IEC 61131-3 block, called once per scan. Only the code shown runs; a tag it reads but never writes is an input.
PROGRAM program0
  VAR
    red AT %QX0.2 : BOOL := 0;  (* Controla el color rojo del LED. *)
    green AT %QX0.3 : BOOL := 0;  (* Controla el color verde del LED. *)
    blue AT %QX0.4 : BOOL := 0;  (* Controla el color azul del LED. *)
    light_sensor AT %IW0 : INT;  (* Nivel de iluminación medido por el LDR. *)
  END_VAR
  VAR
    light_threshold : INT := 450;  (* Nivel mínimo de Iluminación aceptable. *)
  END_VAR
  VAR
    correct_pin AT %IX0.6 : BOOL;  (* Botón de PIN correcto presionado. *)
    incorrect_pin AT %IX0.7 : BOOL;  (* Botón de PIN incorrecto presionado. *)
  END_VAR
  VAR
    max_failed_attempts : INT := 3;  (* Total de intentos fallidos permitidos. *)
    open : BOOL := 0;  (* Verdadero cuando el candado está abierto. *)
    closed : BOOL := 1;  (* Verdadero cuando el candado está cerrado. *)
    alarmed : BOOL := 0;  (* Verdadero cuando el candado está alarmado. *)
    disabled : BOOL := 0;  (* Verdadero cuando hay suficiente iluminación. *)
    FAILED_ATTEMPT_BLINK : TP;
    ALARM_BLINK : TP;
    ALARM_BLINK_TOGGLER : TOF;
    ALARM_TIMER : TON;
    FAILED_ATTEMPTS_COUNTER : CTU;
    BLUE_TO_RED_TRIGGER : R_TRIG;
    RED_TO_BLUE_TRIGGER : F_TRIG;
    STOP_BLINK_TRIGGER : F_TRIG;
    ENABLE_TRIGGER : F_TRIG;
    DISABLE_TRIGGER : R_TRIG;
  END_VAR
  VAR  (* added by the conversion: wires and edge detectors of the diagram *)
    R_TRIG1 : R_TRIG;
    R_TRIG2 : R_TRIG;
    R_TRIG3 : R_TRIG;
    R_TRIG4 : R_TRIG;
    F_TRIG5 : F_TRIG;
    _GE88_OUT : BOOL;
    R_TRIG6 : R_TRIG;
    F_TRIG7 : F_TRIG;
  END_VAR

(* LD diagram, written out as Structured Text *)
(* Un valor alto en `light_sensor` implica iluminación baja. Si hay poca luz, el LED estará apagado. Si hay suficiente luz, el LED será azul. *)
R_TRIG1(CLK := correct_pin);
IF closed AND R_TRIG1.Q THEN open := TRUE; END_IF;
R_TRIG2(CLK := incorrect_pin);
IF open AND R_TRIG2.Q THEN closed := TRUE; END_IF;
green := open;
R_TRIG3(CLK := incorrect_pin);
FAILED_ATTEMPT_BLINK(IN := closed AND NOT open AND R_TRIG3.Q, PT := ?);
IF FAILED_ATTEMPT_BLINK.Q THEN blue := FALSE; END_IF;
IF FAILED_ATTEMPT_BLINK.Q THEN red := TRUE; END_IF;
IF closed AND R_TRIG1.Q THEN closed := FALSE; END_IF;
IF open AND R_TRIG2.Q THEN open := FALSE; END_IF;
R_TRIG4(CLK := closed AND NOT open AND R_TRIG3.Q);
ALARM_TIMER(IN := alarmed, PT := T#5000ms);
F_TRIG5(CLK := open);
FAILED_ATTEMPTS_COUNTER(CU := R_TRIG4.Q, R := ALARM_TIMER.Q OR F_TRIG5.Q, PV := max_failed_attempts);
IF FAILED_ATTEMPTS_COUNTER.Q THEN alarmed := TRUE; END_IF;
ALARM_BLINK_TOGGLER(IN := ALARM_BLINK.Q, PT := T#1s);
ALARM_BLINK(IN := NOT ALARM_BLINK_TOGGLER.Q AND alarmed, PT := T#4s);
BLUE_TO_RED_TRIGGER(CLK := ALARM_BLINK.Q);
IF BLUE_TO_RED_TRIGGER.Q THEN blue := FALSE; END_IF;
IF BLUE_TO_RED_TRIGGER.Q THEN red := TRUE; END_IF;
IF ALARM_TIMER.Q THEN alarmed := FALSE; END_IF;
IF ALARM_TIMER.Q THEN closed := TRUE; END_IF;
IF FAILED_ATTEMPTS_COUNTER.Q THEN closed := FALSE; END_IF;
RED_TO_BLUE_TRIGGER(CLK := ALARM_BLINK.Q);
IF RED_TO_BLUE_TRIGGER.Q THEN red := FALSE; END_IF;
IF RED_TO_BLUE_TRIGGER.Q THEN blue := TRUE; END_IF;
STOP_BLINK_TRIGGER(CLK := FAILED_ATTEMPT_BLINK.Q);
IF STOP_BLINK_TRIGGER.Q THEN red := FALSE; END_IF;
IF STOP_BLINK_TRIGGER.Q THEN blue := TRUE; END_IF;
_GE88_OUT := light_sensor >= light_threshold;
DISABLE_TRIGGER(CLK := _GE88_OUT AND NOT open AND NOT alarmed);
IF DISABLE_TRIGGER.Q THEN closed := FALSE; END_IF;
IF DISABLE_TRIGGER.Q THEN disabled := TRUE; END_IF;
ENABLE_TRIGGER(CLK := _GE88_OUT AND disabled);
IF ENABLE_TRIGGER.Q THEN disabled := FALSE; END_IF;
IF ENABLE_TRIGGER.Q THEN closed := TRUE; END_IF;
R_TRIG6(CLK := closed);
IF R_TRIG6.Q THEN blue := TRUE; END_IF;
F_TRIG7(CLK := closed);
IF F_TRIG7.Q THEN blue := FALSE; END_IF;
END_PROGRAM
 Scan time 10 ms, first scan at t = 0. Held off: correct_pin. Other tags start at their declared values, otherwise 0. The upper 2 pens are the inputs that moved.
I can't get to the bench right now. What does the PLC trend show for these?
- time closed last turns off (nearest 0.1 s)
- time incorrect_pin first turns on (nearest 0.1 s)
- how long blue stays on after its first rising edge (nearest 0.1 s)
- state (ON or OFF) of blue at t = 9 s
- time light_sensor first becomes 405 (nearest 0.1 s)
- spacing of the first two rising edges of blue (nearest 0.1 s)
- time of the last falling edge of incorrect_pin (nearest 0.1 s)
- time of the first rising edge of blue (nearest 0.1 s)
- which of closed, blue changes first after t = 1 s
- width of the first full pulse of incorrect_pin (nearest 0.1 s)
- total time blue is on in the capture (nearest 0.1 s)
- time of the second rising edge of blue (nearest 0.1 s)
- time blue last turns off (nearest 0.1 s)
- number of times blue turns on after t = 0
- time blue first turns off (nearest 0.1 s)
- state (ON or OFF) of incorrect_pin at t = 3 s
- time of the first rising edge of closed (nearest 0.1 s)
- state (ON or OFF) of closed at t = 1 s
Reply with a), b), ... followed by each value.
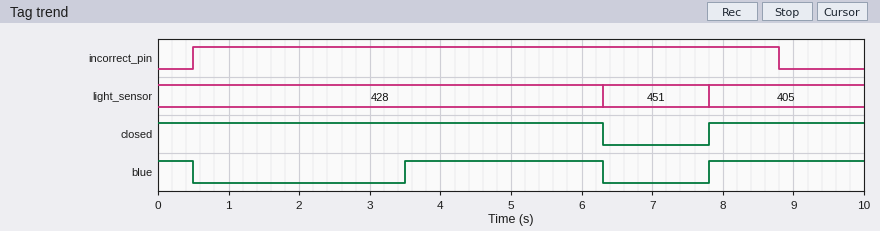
a) 6.3 s
b) 0.5 s
c) 2.8 s
d) ON
e) 7.8 s
f) 4.3 s
g) 8.8 s
h) 3.5 s
i) blue
j) 8.3 s
k) 5.5 s
l) 7.8 s
m) 6.3 s
n) 2
o) 0.5 s
p) ON
q) 7.8 s
r) ON
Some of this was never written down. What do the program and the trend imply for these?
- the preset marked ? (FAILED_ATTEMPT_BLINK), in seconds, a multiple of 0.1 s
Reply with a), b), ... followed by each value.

a) 3.0 s
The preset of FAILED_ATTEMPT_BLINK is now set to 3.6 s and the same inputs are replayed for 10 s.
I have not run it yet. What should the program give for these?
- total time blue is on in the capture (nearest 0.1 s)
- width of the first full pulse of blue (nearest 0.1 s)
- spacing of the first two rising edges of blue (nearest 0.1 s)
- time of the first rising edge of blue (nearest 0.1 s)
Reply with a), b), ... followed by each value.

a) 4.9 s
b) 2.2 s
c) 3.7 s
d) 4.1 s
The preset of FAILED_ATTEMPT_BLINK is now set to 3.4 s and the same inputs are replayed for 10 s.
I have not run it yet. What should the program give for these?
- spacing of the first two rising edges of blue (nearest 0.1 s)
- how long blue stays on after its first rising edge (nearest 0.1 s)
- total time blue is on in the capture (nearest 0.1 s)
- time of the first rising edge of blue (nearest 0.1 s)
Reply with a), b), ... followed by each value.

a) 3.9 s
b) 2.4 s
c) 5.1 s
d) 3.9 s
